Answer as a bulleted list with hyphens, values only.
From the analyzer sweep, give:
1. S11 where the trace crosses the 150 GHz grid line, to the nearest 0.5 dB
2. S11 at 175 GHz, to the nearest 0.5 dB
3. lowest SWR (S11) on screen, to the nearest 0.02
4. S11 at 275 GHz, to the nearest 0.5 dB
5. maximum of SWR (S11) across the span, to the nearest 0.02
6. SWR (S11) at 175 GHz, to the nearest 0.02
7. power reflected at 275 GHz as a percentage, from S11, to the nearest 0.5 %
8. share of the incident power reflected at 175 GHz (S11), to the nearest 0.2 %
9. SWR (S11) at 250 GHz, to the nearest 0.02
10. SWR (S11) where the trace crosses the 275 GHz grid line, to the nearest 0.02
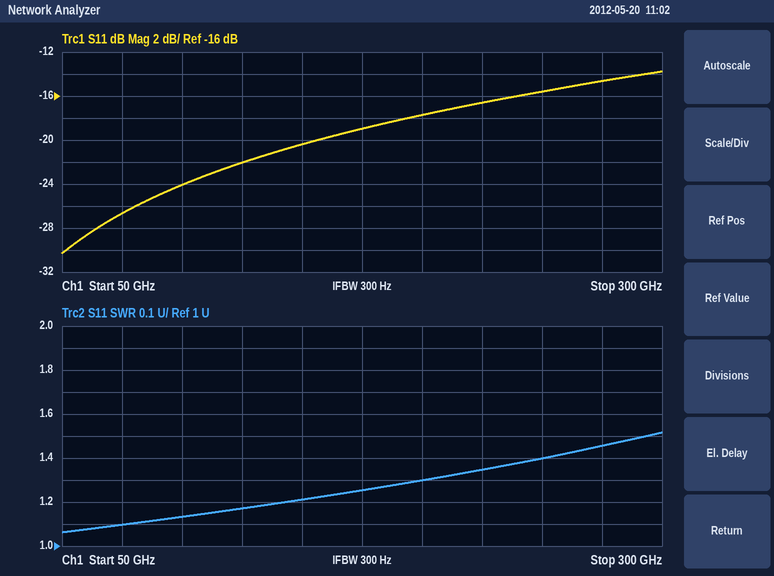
- -20.5 dB
- -19.0 dB
- 1.06
- -14.5 dB
- 1.52
- 1.26
- 3.5 %
- 1.2 %
- 1.40
- 1.46
